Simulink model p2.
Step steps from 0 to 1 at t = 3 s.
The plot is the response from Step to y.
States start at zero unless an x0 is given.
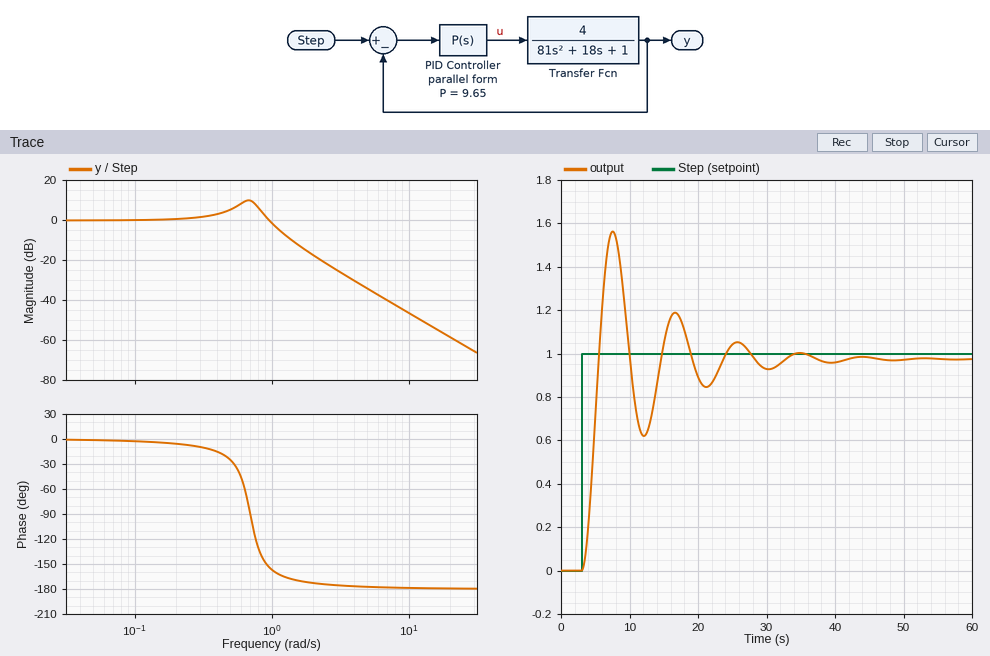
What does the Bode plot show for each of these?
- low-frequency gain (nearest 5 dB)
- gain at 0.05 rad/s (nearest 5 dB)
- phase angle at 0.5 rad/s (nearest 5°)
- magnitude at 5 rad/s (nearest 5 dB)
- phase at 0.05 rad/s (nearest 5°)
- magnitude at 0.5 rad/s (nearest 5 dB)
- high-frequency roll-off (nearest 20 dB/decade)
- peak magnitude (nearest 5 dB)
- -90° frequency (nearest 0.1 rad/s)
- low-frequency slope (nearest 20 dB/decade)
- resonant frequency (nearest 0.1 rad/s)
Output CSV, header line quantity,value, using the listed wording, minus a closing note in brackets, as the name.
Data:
quantity,value
low-frequency gain,0 dB
gain at 0.05 rad/s,0 dB
phase angle at 0.5 rad/s,-25°
magnitude at 5 rad/s,-35 dB
phase at 0.05 rad/s,0°
magnitude at 0.5 rad/s,5 dB
high-frequency roll-off,-40 dB/decade
peak magnitude,10 dB
-90° frequency,0.7 rad/s
low-frequency slope,0 dB/decade
resonant frequency,0.7 rad/s
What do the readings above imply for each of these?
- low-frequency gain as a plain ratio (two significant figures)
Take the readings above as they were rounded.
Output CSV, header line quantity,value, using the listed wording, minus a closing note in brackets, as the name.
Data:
quantity,value
low-frequency gain as a plain ratio,1.0
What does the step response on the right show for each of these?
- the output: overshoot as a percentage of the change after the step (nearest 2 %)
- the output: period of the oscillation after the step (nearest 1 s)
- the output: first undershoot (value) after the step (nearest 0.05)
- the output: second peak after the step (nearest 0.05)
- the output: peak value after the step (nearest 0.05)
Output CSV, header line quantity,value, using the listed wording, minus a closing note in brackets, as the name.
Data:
quantity,value
the output: overshoot as a percentage of the change after the step,60 %
the output: period of the oscillation after the step,9 s
the output: first undershoot (value) after the step,0.60
the output: second peak after the step,1.20
the output: peak value after the step,1.55
